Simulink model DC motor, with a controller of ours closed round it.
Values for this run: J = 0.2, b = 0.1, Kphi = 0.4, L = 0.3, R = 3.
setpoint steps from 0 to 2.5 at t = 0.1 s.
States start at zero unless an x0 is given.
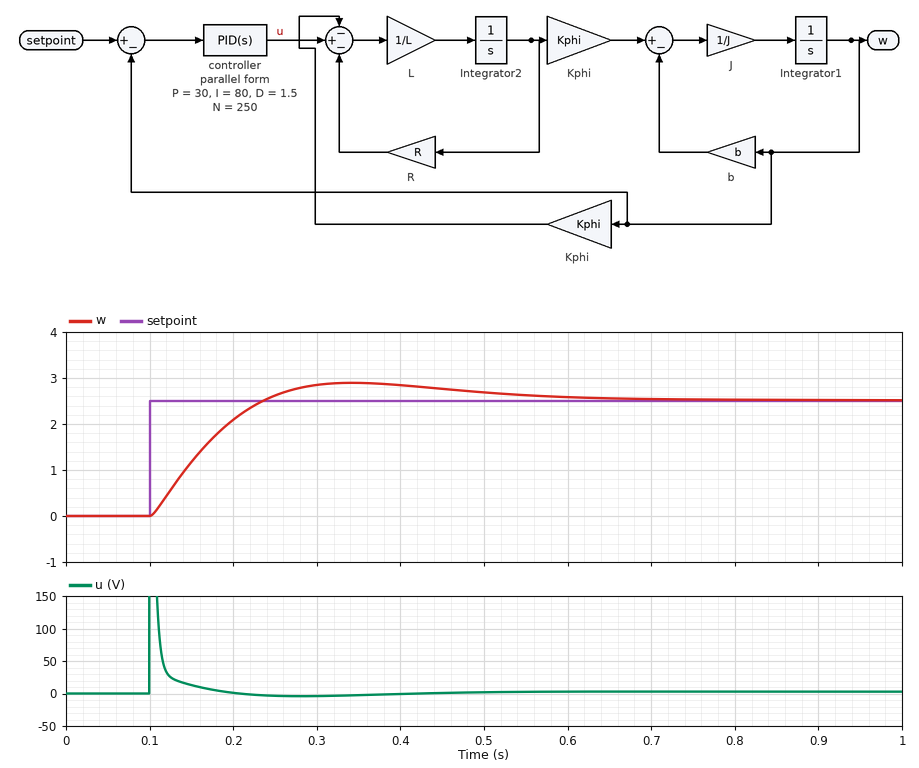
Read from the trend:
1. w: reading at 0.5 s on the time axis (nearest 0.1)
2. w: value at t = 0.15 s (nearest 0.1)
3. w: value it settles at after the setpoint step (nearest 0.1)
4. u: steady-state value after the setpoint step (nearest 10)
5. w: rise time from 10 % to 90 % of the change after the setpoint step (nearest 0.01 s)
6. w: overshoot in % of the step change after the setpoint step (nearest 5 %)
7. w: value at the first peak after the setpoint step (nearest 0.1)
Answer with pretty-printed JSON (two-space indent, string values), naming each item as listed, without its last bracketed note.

{
  "w: reading at 0.5 s on the time axis": "2.7",
  "w: value at t = 0.15 s": "1.2",
  "w: value it settles at after the setpoint step": "2.5",
  "u: steady-state value after the setpoint step": "0",
  "w: rise time from 10 % to 90 % of the change after the setpoint step": "0.10 s",
  "w: overshoot in % of the step change after the setpoint step": "15 %",
  "w: value at the first peak after the setpoint step": "2.9"
}
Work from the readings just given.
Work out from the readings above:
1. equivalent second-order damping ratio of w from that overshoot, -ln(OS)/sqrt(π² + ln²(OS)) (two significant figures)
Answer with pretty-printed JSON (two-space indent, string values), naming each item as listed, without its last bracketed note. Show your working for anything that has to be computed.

{
  "equivalent second-order damping ratio of w from that overshoot, -ln(OS)/sqrt(π² + ln²(OS))": "ln(0.15) = -1.897; 1.897 / sqrt(9.870 + 3.599) = 0.52"
}
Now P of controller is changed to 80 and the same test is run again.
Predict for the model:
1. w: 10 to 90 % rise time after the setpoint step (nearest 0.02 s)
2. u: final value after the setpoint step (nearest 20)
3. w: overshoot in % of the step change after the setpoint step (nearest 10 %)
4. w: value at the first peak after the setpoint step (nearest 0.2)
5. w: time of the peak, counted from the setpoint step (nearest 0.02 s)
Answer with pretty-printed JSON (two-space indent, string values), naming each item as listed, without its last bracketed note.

{
  "w: 10 to 90 % rise time after the setpoint step": "0.06 s",
  "u: final value after the setpoint step": "0",
  "w: overshoot in % of the step change after the setpoint step": "30 %",
  "w: value at the first peak after the setpoint step": "3.2",
  "w: time of the peak, counted from the setpoint step": "0.12 s"
}
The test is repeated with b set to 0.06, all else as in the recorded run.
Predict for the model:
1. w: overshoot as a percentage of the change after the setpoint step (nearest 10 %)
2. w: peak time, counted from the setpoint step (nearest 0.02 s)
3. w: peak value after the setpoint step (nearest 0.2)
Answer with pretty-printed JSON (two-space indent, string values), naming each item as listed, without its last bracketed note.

{
  "w: overshoot as a percentage of the change after the setpoint step": "20 %",
  "w: peak time, counted from the setpoint step": "0.24 s",
  "w: peak value after the setpoint step": "3.0"
}
